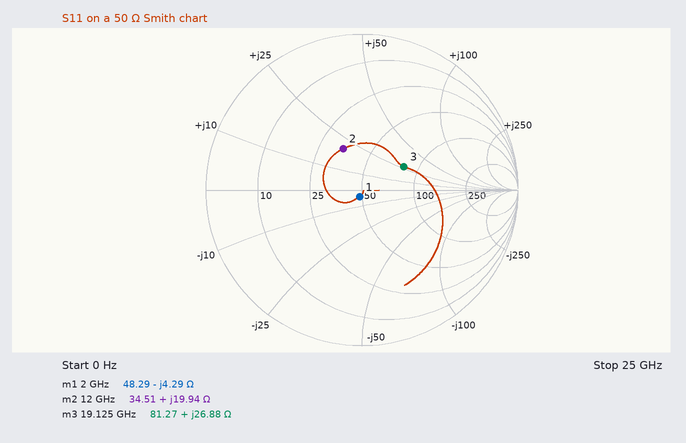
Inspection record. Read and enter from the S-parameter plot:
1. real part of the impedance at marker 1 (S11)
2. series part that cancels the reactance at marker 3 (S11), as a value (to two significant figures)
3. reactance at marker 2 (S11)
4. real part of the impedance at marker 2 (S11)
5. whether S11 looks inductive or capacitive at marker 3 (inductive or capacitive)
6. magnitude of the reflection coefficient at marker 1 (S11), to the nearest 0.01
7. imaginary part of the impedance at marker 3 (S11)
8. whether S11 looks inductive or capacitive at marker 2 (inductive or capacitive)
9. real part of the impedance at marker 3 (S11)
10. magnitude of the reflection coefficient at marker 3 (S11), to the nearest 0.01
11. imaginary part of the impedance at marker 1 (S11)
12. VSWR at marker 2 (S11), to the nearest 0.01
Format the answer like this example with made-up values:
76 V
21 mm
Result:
48.29 Ω
310 fF
+19.94 Ω
34.51 Ω
inductive
0.05
+26.88 Ω
inductive
81.27 Ω
0.31
-4.29 Ω
1.82
